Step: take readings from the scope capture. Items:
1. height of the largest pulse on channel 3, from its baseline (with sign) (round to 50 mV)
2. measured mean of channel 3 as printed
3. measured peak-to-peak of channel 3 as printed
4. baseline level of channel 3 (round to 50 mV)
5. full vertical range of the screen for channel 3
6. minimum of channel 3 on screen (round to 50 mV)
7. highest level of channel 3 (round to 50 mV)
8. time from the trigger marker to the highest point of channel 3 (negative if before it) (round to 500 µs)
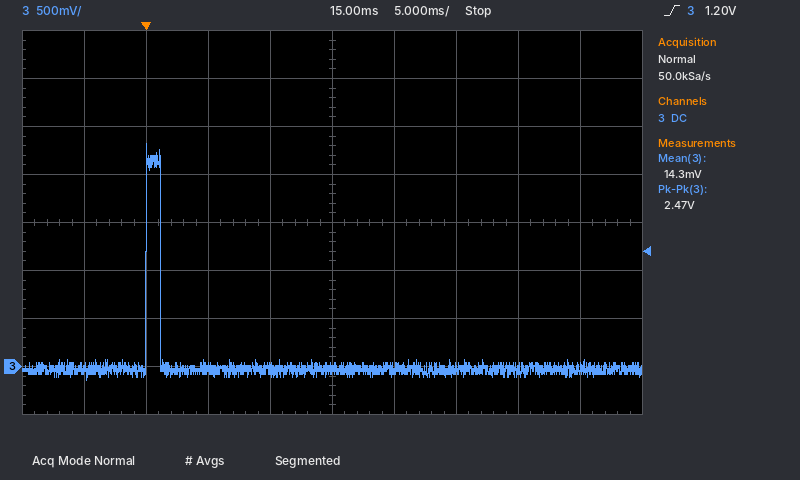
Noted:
+2.35 V
14.3 mV
2.47 V
-50 mV
4 V
-150 mV
2.30 V
0.0 ms
